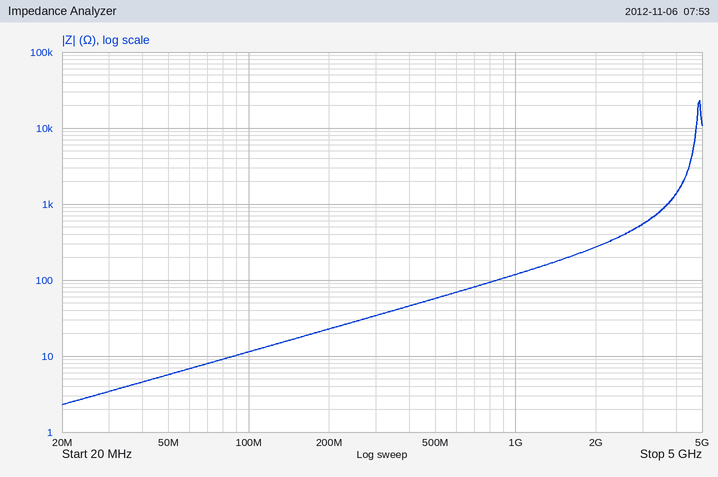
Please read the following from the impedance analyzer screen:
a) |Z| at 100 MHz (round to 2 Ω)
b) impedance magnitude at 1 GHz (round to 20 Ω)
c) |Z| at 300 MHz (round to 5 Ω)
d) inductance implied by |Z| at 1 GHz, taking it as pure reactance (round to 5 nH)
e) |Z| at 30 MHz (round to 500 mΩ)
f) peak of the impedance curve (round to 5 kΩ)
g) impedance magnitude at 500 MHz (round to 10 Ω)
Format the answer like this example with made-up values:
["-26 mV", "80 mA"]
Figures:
["12 Ω", "120 Ω", "35 Ω", "20 nH", "3.5 Ω", "25 kΩ", "60 Ω"]
